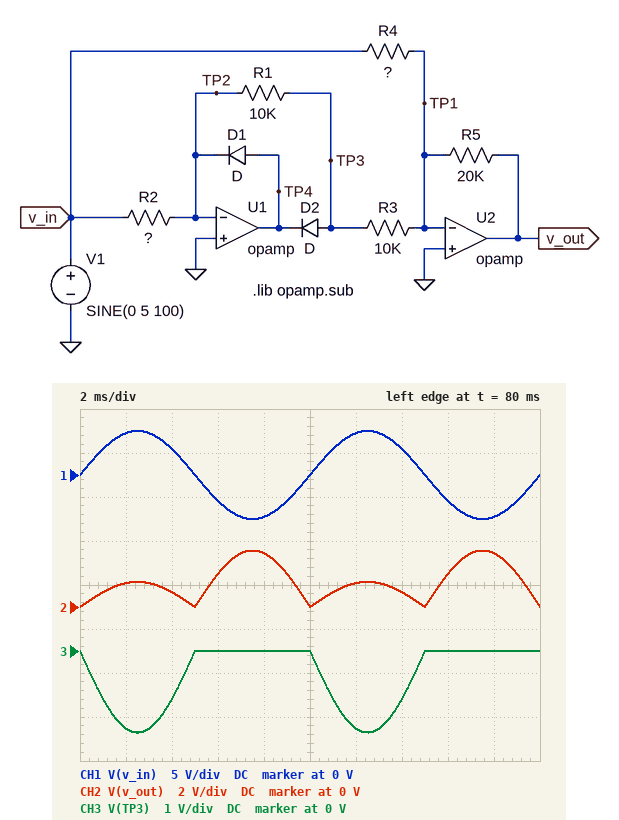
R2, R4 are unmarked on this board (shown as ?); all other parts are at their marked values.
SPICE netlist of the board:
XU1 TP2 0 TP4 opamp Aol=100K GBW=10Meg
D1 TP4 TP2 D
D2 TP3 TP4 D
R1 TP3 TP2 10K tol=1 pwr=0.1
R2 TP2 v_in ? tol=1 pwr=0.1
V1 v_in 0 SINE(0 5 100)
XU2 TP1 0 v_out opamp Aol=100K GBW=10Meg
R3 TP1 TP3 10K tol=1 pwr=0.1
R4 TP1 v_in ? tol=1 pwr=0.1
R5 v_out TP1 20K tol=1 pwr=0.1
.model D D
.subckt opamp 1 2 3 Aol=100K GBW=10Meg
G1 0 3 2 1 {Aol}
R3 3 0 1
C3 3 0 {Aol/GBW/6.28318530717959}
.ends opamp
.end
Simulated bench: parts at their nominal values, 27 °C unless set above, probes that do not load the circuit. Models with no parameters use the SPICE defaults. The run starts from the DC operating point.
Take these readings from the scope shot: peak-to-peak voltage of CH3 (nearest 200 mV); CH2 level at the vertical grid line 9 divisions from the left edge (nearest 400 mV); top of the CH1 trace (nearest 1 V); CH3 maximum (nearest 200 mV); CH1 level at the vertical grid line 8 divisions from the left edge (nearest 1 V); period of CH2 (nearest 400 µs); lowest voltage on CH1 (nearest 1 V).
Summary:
1.8 V
2.4 V
5 V
0 V
-3 V
10.0 ms
-5 V
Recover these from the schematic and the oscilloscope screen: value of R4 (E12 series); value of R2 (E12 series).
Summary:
39 kΩ
27 kΩ
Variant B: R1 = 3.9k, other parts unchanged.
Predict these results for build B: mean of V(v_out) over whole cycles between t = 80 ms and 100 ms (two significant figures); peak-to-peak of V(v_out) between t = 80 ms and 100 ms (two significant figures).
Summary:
460 mV
3.7 V
